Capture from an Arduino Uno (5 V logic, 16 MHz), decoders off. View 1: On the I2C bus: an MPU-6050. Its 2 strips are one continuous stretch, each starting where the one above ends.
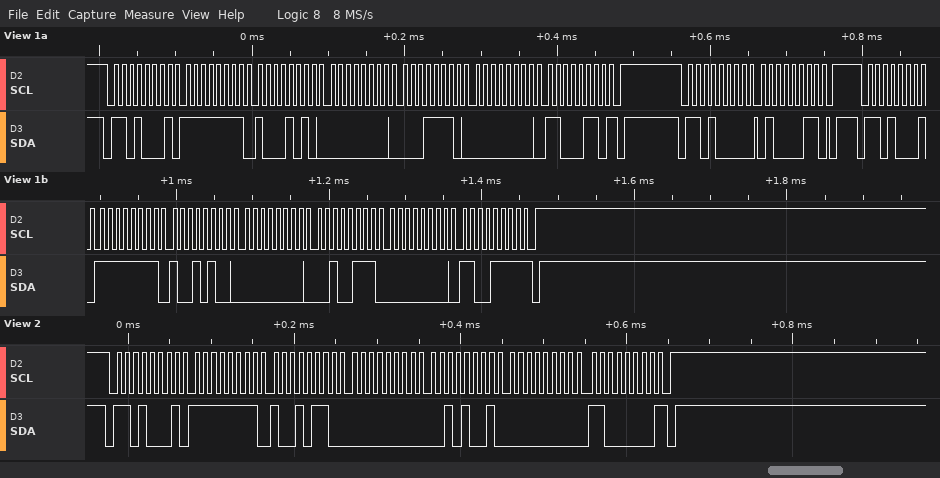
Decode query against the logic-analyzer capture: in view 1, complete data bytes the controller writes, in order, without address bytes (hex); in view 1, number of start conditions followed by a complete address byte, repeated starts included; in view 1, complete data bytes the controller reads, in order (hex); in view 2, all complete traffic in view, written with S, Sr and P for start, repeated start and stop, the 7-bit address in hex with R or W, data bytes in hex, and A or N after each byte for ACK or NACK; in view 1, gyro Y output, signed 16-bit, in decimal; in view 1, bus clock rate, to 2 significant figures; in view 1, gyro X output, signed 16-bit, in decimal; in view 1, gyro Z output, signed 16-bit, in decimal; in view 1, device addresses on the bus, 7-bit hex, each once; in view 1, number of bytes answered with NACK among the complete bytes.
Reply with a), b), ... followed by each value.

a) 43
b) 3
c) FF 8A 00 1E 00 C6 FF 94 00 27 00 CF
d) S 68R A FF A 96 A 00 A 29 A 00 A C0 N P
e) 39
f) 100 kHz
g) -108
h) 207
i) 0x68
j) 2
